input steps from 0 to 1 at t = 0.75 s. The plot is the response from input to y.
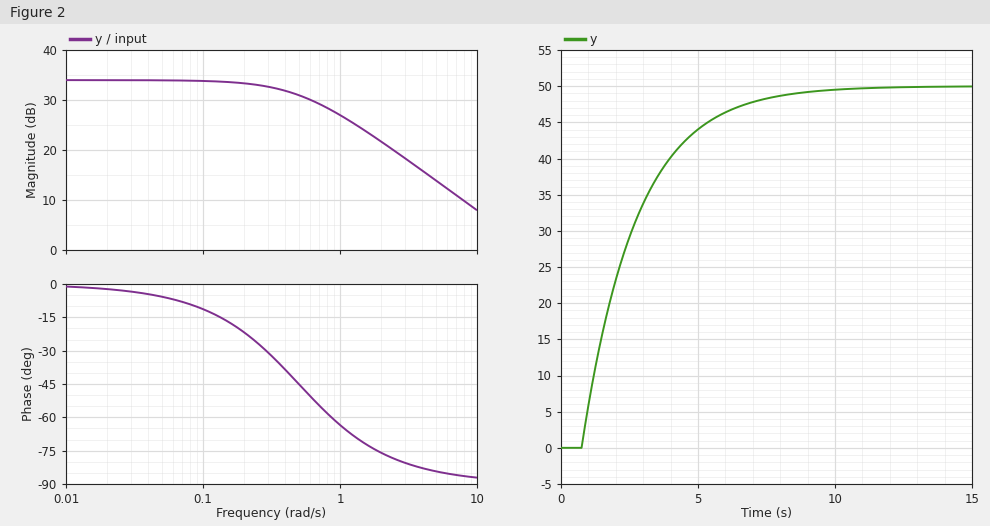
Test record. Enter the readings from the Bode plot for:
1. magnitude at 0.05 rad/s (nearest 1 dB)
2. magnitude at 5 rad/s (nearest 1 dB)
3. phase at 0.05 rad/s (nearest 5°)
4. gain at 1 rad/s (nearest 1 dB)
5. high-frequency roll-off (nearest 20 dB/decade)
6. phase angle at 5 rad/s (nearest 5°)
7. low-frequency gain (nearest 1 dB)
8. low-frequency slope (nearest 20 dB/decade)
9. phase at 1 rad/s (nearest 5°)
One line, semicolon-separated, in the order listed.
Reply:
34 dB; 14 dB; -5°; 27 dB; -20 dB/decade; -85°; 34 dB; 0 dB/decade; -65°
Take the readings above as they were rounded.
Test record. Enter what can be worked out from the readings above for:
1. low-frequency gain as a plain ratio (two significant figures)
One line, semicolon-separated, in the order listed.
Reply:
50
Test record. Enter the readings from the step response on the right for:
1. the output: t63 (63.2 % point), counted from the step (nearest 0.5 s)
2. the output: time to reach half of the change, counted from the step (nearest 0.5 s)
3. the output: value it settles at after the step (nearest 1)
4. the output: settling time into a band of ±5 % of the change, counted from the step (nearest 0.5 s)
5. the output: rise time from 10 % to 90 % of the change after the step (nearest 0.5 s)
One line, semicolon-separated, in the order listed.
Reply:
2.0 s; 1.5 s; 50; 6.0 s; 4.5 s
